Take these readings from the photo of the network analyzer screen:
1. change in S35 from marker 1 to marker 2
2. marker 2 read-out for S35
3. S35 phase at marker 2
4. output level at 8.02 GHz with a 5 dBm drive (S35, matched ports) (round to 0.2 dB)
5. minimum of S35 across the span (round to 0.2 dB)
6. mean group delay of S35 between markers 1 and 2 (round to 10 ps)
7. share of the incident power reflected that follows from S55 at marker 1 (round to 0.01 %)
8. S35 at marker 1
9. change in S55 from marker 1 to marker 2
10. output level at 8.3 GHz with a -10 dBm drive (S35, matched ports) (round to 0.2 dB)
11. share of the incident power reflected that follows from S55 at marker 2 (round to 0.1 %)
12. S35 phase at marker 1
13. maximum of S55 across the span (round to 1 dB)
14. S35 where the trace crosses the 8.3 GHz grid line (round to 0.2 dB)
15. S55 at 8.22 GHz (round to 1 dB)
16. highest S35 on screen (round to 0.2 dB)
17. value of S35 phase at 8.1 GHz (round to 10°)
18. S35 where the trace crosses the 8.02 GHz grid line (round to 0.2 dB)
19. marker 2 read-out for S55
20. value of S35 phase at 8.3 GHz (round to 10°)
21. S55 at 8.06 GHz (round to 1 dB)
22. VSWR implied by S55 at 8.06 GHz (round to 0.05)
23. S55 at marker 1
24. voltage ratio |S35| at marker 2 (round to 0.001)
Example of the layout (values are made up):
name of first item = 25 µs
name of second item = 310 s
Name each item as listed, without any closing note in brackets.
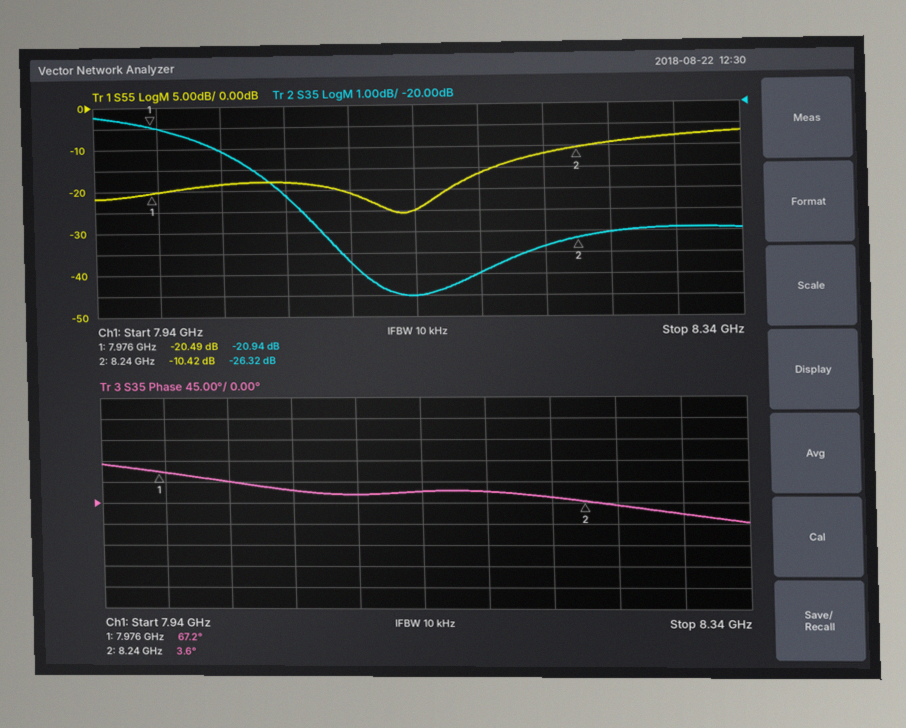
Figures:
change in S35 from marker 1 to marker 2 = -5.38 dB
marker 2 read-out for S35 = -26.32 dB
S35 phase at marker 2 = 3.6°
output level at 8.02 GHz with a 5 dBm drive (S35, matched ports) = -17.2 dBm
minimum of S35 across the span = -29.0 dB
mean group delay of S35 between markers 1 and 2 = 670 ps
share of the incident power reflected that follows from S55 at marker 1 = 0.89 %
S35 at marker 1 = -20.94 dB
change in S55 from marker 1 to marker 2 = 10.07 dB
output level at 8.3 GHz with a -10 dBm drive (S35, matched ports) = -35.8 dBm
share of the incident power reflected that follows from S55 at marker 2 = 9.1 %
S35 phase at marker 1 = 67.2°
maximum of S55 across the span = -7 dB
S35 where the trace crosses the 8.3 GHz grid line = -25.8 dB
S55 at 8.22 GHz = -12 dB
highest S35 on screen = -20.4 dB
value of S35 phase at 8.1 GHz = 20°
S35 where the trace crosses the 8.02 GHz grid line = -22.2 dB
marker 2 read-out for S55 = -10.42 dB
value of S35 phase at 8.3 GHz = -20°
S55 at 8.06 GHz = -18 dB
VSWR implied by S55 at 8.06 GHz = 1.30
S55 at marker 1 = -20.49 dB
voltage ratio |S35| at marker 2 = 0.048
